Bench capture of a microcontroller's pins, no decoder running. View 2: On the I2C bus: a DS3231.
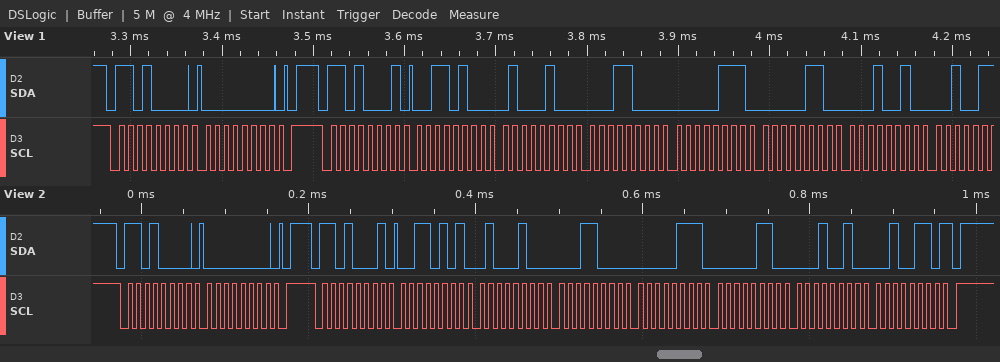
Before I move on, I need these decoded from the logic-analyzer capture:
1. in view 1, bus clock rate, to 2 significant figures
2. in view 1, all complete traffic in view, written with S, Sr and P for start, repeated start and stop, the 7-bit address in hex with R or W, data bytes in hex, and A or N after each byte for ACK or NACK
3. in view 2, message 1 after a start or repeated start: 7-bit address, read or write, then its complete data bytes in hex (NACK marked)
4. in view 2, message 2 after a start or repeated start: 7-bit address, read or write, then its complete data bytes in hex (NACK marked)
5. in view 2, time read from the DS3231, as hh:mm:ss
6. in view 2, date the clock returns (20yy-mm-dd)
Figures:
100 kHz
S 68W A 00 A P S 68R A 34 A 44 A 18 A 07 A 06 A 12 A
0x68 write: 00
0x68 read: 35 44 18 07 06 12 26 NACK
18:44:35
2026-12-06
